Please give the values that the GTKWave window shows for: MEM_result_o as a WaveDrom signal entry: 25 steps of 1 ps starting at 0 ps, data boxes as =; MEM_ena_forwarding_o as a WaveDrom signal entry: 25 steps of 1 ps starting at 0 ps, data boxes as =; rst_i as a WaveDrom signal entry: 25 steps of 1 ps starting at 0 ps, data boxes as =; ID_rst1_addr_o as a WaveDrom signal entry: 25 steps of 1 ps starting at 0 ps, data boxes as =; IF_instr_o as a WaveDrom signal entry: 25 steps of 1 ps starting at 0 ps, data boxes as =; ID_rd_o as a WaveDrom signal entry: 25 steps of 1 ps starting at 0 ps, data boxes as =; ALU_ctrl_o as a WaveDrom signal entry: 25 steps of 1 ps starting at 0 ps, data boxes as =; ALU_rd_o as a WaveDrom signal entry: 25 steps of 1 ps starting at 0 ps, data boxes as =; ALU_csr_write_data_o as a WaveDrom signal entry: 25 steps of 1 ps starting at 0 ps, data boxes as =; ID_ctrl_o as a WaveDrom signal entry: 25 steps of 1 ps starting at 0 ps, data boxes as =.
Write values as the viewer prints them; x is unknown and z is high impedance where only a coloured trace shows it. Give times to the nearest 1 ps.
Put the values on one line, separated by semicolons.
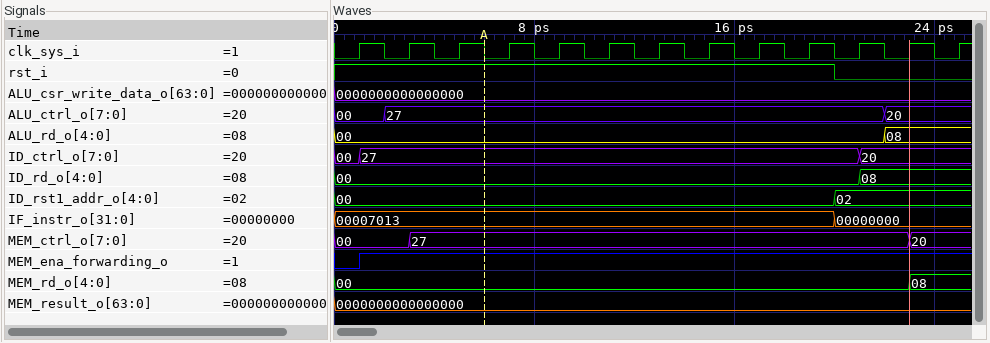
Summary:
{name: 'MEM_result_o', wave: '=........................', data: '0000000000000000'}; {name: 'MEM_ena_forwarding_o', wave: '01.......................'}; {name: 'rst_i', wave: '1...................0....'}; {name: 'ID_rst1_addr_o', wave: '=...................=....', data: '00 02'}; {name: 'IF_instr_o', wave: '=...................=....', data: '00007013 00000000'}; {name: 'ID_rd_o', wave: '=....................=...', data: '00 08'}; {name: 'ALU_ctrl_o', wave: '=.=...................=..', data: '00 27 20'}; {name: 'ALU_rd_o', wave: '=.....................=..', data: '00 08'}; {name: 'ALU_csr_write_data_o', wave: '=........................', data: '0000000000000000'}; {name: 'ID_ctrl_o', wave: '==...................=...', data: '00 27 20'}
